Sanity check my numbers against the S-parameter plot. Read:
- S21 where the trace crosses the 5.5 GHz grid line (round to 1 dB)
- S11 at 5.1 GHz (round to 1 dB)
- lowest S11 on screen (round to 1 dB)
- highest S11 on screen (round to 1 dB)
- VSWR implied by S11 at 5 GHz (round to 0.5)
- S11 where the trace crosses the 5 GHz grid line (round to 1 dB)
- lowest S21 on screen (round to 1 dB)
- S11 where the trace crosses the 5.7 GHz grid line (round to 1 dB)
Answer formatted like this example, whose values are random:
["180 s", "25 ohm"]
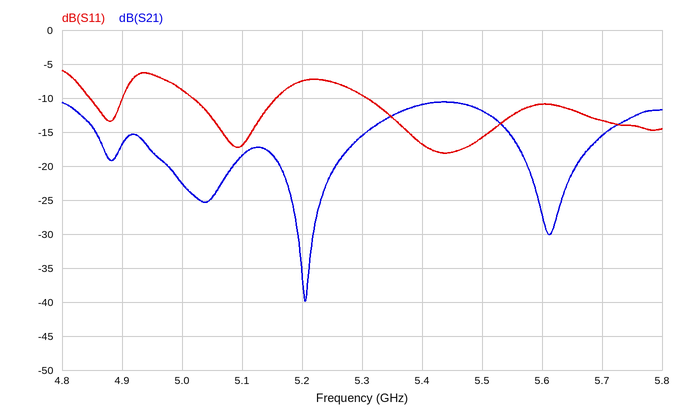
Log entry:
["-12 dB", "-17 dB", "-18 dB", "-6 dB", "2.0", "-9 dB", "-40 dB", "-13 dB"]
